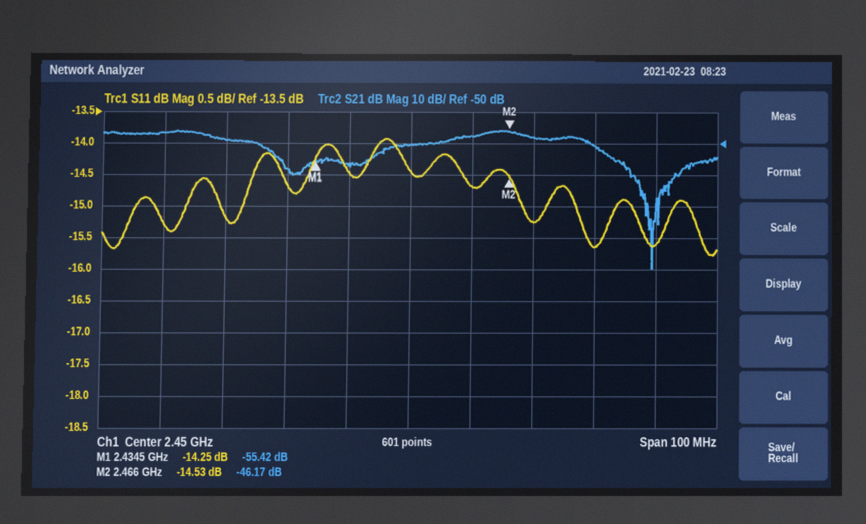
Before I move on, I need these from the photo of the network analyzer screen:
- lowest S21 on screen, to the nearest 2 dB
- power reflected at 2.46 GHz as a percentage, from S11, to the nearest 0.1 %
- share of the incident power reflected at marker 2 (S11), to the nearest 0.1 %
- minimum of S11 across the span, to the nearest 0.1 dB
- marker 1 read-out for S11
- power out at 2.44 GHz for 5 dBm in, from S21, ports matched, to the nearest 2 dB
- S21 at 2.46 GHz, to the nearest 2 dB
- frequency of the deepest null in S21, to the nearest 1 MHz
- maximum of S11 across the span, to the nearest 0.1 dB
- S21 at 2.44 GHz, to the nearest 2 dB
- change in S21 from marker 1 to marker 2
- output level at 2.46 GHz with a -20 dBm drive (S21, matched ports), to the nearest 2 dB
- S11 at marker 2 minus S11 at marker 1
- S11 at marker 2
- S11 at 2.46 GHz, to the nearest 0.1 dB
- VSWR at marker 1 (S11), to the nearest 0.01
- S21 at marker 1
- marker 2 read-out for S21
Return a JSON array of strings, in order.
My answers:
["-90 dB", "3.4 %", "3.5 %", "-15.8 dB", "-14.25 dB", "-52 dBm", "-48 dB", "2.489 GHz", "-13.9 dB", "-56 dB", "9.25 dB", "-68 dBm", "-0.28 dB", "-14.53 dB", "-14.7 dB", "1.48", "-55.42 dB", "-46.17 dB"]
